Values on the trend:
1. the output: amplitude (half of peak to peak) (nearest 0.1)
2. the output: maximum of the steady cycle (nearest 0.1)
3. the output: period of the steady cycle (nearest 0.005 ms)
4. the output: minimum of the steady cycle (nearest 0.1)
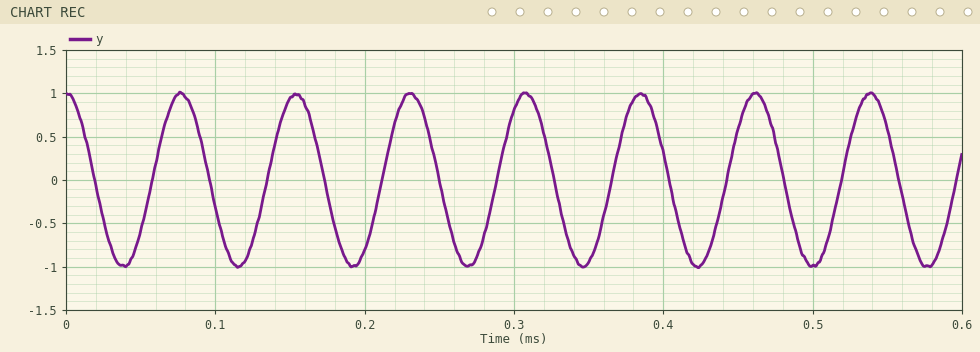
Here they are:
1.0
1.0
0.075 ms
-1.0
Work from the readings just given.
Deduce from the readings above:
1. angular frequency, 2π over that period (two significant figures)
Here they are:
84 rad/ms
